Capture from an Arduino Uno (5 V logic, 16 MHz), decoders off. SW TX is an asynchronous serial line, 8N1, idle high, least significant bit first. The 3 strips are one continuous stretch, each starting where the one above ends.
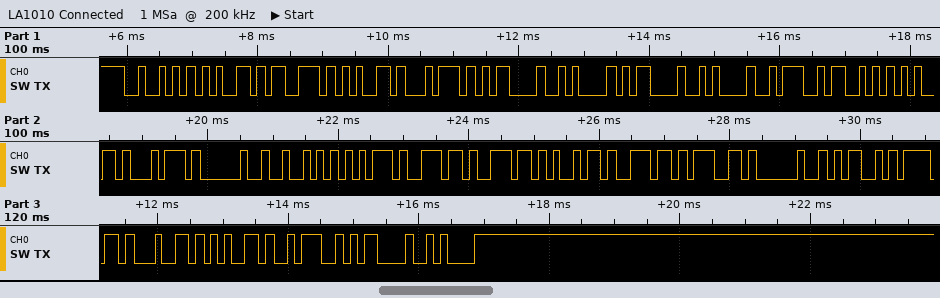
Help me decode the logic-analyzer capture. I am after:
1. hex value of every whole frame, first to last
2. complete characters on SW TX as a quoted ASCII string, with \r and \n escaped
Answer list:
52 65 73 65 74 0D 0A 0D 0A 3A 53 65 74 20 52 75 6E 6E 69 6E 67 20 4D 6F 64 65 3A 0D 0A
"Reset\r\n\r\n:Set Running Mode:\r\n"
